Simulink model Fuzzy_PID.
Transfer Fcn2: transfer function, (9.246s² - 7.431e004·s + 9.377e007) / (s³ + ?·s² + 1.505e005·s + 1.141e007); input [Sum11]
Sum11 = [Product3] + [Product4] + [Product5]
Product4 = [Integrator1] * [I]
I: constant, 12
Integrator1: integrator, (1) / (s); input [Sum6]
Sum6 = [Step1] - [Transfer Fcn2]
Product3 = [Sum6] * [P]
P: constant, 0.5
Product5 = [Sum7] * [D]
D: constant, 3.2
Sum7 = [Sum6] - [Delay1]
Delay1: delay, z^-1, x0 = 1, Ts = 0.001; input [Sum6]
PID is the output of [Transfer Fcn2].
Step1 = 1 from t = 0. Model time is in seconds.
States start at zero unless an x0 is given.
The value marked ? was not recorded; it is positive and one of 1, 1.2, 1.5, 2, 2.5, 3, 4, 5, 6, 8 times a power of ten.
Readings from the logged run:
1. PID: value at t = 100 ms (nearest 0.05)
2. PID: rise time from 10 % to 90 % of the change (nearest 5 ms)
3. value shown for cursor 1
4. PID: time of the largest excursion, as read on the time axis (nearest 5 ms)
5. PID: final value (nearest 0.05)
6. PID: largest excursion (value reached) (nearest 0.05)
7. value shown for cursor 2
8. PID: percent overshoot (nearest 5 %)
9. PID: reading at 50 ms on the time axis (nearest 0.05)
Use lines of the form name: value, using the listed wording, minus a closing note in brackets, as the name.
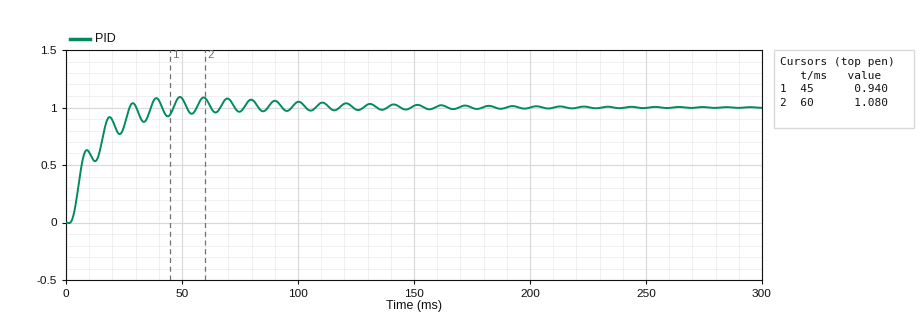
PID: value at t = 100 ms: 1.05
PID: rise time from 10 % to 90 % of the change: 15 ms
value shown for cursor 1: 0.940
PID: time of the largest excursion, as read on the time axis: 50 ms
PID: final value: 1.00
PID: largest excursion (value reached): 1.10
value shown for cursor 2: 1.080
PID: percent overshoot: 10 %
PID: reading at 50 ms on the time axis: 1.10
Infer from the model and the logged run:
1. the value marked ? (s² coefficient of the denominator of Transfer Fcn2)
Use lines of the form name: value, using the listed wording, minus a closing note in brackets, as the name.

the value marked ?: 800
